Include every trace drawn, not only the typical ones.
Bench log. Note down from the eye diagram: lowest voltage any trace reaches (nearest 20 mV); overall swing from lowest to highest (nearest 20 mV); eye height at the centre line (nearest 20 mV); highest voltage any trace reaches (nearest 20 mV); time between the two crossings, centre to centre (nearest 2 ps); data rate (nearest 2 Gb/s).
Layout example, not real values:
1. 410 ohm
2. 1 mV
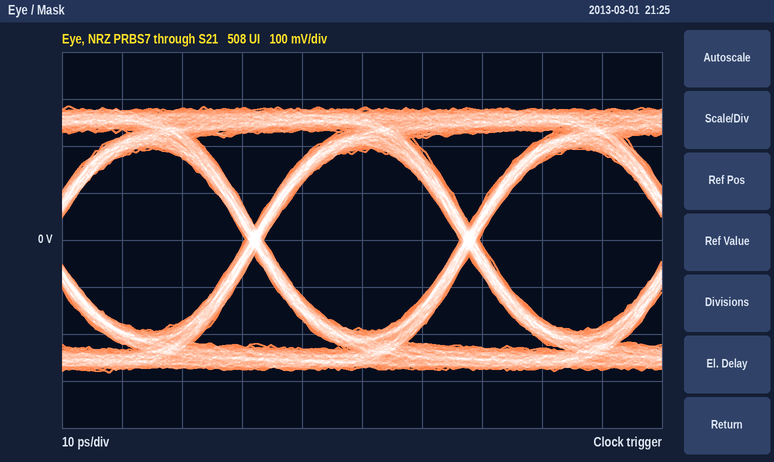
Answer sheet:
1. -280 mV
2. 560 mV
3. 380 mV
4. 280 mV
5. 36 ps
6. 28 Gb/s
